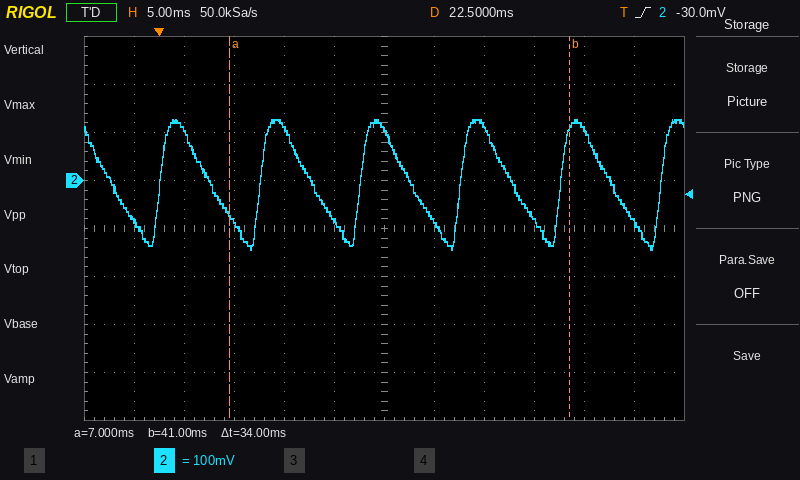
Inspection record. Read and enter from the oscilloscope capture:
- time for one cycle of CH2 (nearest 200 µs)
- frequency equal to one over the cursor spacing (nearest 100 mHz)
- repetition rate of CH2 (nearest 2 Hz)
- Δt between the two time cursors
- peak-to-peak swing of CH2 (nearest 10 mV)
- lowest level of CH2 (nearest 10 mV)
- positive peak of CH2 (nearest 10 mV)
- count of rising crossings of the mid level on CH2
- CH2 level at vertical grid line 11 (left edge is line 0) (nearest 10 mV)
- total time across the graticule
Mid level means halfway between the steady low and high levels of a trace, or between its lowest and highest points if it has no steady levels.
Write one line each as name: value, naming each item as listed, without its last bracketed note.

time for one cycle of CH2: 10.0 ms
frequency equal to one over the cursor spacing: 29.4 Hz
repetition rate of CH2: 100 Hz
Δt between the two time cursors: 34 ms
peak-to-peak swing of CH2: 270 mV
lowest level of CH2: -140 mV
positive peak of CH2: 130 mV
count of rising crossings of the mid level on CH2: 6
CH2 level at vertical grid line 11 (left edge is line 0): -90 mV
total time across the graticule: 60 ms
